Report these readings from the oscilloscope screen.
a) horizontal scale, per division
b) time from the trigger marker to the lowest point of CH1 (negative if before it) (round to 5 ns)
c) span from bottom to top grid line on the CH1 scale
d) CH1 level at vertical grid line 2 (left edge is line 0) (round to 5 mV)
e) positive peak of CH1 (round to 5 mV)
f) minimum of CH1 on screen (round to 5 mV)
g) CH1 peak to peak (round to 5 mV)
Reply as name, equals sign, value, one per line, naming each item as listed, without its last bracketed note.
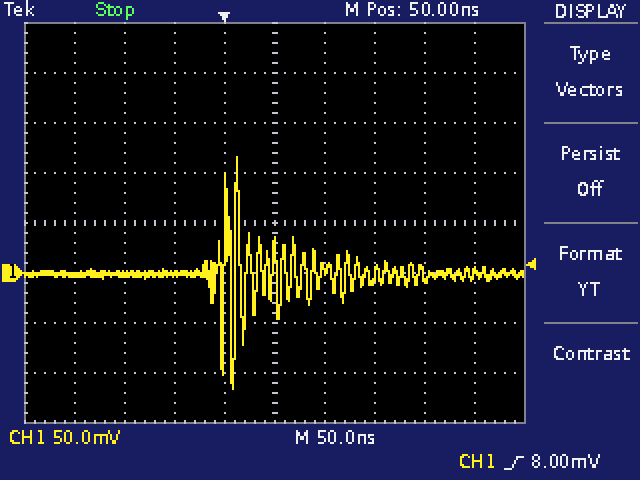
horizontal scale, per division = 50 ns
time from the trigger marker to the lowest point of CH1 (negative if before it) = +10 ns
span from bottom to top grid line on the CH1 scale = 400 mV
CH1 level at vertical grid line 2 (left edge is line 0) = 0 mV
positive peak of CH1 = 115 mV
minimum of CH1 on screen = -115 mV
CH1 peak to peak = 230 mV
